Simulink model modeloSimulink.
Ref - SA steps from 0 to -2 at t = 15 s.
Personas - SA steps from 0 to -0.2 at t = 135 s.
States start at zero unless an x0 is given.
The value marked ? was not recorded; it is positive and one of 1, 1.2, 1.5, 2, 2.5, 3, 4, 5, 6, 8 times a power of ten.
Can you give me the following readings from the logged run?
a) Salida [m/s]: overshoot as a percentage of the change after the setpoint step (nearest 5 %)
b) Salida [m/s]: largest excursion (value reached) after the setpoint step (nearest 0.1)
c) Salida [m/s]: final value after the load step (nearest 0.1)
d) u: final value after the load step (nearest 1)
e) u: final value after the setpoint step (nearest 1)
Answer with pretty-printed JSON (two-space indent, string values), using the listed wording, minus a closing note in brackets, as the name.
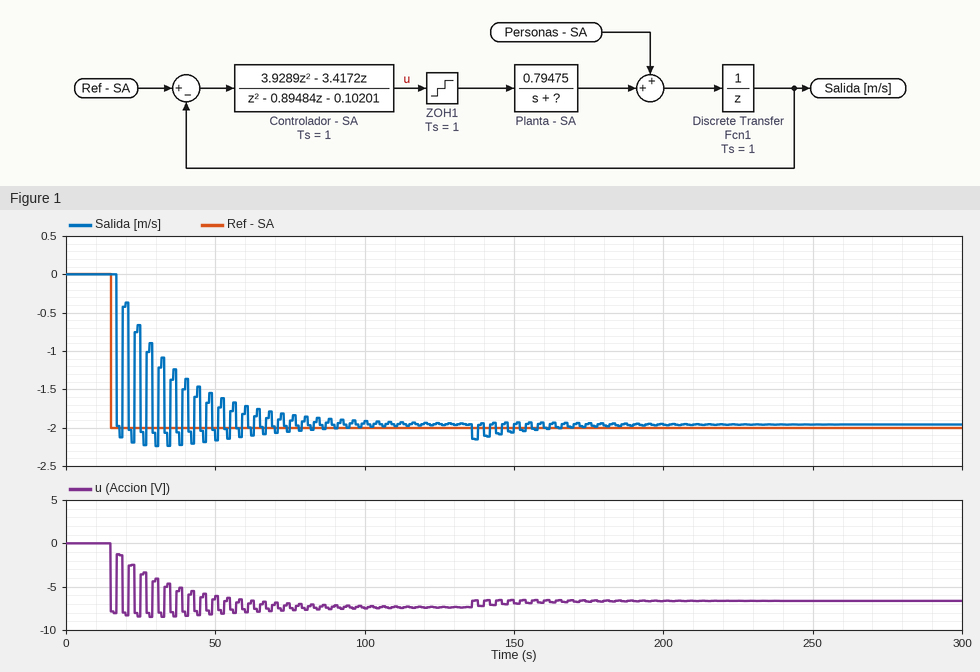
{
  "Salida [m/s]: overshoot as a percentage of the change after the setpoint step": "15 %",
  "Salida [m/s]: largest excursion (value reached) after the setpoint step": "-2.2",
  "Salida [m/s]: final value after the load step": "-2.0",
  "u: final value after the load step": "-7",
  "u: final value after the setpoint step": "-7"
}
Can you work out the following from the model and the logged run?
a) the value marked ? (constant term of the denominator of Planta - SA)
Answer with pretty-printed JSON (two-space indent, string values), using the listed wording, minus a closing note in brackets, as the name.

{
  "the value marked ?": "3"
}
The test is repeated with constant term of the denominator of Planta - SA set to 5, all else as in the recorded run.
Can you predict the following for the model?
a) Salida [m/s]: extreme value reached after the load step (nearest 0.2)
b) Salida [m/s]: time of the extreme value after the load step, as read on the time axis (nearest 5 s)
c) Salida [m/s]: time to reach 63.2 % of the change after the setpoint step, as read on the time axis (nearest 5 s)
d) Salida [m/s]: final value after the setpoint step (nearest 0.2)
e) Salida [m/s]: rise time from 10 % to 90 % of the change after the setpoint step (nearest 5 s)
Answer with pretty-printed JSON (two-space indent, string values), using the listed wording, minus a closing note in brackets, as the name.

{
  "Salida [m/s]: extreme value reached after the load step": "-2.2",
  "Salida [m/s]: time of the extreme value after the load step, as read on the time axis": "135 s",
  "Salida [m/s]: time to reach 63.2 % of the change after the setpoint step, as read on the time axis": "15 s",
  "Salida [m/s]: final value after the setpoint step": "-2.0",
  "Salida [m/s]: rise time from 10 % to 90 % of the change after the setpoint step": "35 s"
}
